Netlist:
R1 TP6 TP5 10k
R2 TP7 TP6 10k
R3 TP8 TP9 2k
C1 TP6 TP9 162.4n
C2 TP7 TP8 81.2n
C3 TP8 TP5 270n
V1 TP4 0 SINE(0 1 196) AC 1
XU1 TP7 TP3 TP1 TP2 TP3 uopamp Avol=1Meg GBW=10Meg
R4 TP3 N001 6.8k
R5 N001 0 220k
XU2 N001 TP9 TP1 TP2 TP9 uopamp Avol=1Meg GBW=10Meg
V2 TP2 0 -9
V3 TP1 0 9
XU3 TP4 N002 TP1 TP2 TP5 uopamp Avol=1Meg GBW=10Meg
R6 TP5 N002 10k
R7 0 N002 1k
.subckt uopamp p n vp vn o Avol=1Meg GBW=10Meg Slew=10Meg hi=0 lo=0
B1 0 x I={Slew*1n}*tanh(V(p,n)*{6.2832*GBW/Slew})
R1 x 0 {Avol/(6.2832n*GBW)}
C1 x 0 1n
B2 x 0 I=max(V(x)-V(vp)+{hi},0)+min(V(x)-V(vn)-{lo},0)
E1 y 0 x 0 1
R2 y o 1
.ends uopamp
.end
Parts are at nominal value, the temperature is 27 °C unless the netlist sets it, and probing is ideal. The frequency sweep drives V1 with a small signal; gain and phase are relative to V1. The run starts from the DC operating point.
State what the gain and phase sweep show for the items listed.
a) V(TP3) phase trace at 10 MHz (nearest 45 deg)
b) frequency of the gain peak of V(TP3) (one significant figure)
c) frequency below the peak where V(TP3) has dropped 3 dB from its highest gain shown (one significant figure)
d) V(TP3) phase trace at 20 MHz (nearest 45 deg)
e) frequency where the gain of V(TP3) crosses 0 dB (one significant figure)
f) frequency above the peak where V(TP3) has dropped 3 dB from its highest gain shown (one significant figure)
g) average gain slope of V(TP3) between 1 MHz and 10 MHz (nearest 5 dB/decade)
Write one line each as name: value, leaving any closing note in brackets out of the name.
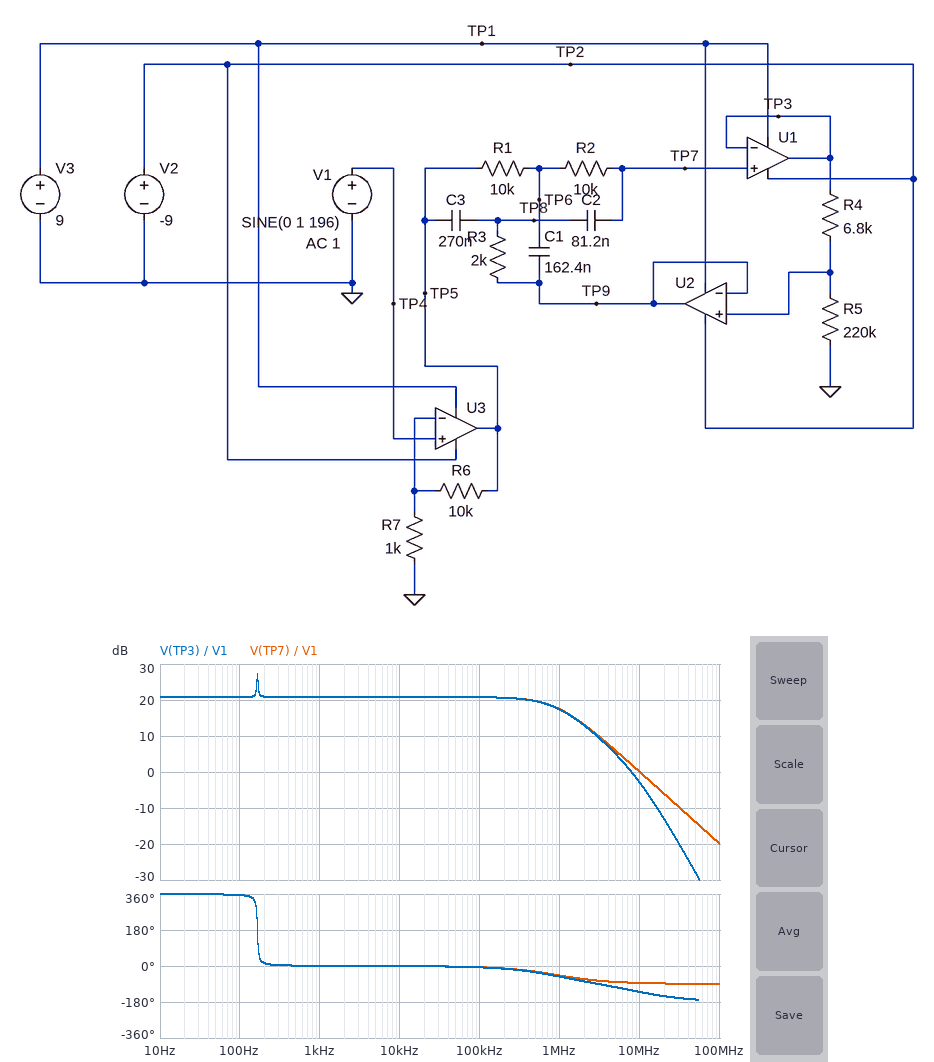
V(TP3) phase trace at 10 MHz: -135 deg
frequency of the gain peak of V(TP3): 200 Hz
frequency below the peak where V(TP3) has dropped 3 dB from its highest gain shown: 200 Hz
V(TP3) phase trace at 20 MHz: -135 deg
frequency where the gain of V(TP3) crosses 0 dB: 8 MHz
frequency above the peak where V(TP3) has dropped 3 dB from its highest gain shown: 200 Hz
average gain slope of V(TP3) between 1 MHz and 10 MHz: -20 dB/decade
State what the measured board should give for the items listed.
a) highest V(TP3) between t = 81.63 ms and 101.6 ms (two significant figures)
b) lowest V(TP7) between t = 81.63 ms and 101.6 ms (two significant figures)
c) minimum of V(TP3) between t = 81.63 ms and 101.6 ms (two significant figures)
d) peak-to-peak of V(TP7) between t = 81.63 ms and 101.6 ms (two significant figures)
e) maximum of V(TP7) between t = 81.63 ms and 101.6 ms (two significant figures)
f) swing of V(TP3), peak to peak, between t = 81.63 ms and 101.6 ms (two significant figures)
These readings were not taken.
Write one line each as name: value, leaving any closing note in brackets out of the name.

highest V(TP3) between t = 81.63 ms and 101.6 ms: 9.0 V
lowest V(TP7) between t = 81.63 ms and 101.6 ms: -9.9 V
minimum of V(TP3) between t = 81.63 ms and 101.6 ms: -9.0 V
peak-to-peak of V(TP7) between t = 81.63 ms and 101.6 ms: 20 V
maximum of V(TP7) between t = 81.63 ms and 101.6 ms: 9.9 V
swing of V(TP3), peak to peak, between t = 81.63 ms and 101.6 ms: 18 V
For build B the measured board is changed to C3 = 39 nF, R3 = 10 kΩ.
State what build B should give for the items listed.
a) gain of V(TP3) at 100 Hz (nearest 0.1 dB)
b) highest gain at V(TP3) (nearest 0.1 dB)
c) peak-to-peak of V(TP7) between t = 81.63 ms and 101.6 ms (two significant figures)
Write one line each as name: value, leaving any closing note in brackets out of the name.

gain of V(TP3) at 100 Hz: 20.7 dB
highest gain at V(TP3): 20.8 dB
peak-to-peak of V(TP7) between t = 81.63 ms and 101.6 ms: 17 V
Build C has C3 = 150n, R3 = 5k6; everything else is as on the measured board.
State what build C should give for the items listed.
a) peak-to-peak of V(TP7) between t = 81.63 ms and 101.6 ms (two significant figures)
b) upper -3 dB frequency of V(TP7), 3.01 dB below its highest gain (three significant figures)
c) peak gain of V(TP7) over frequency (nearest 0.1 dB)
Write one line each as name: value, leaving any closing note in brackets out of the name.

peak-to-peak of V(TP7) between t = 81.63 ms and 101.6 ms: 18 V
upper -3 dB frequency of V(TP7), 3.01 dB below its highest gain: 909 kHz
peak gain of V(TP7) over frequency: 20.8 dB
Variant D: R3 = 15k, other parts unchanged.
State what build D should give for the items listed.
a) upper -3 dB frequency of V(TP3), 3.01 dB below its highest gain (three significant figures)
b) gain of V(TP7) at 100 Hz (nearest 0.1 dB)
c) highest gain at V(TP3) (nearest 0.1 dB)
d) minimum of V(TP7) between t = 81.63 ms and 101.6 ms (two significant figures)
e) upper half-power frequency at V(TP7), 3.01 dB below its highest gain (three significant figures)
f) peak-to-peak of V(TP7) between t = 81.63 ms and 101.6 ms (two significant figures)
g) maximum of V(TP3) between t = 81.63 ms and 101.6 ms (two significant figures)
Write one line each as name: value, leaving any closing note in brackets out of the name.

upper -3 dB frequency of V(TP3), 3.01 dB below its highest gain: 902 kHz
gain of V(TP7) at 100 Hz: 20.4 dB
highest gain at V(TP3): 20.8 dB
minimum of V(TP7) between t = 81.63 ms and 101.6 ms: -8.8 V
upper half-power frequency at V(TP7), 3.01 dB below its highest gain: 909 kHz
peak-to-peak of V(TP7) between t = 81.63 ms and 101.6 ms: 18 V
maximum of V(TP3) between t = 81.63 ms and 101.6 ms: 8.8 V
